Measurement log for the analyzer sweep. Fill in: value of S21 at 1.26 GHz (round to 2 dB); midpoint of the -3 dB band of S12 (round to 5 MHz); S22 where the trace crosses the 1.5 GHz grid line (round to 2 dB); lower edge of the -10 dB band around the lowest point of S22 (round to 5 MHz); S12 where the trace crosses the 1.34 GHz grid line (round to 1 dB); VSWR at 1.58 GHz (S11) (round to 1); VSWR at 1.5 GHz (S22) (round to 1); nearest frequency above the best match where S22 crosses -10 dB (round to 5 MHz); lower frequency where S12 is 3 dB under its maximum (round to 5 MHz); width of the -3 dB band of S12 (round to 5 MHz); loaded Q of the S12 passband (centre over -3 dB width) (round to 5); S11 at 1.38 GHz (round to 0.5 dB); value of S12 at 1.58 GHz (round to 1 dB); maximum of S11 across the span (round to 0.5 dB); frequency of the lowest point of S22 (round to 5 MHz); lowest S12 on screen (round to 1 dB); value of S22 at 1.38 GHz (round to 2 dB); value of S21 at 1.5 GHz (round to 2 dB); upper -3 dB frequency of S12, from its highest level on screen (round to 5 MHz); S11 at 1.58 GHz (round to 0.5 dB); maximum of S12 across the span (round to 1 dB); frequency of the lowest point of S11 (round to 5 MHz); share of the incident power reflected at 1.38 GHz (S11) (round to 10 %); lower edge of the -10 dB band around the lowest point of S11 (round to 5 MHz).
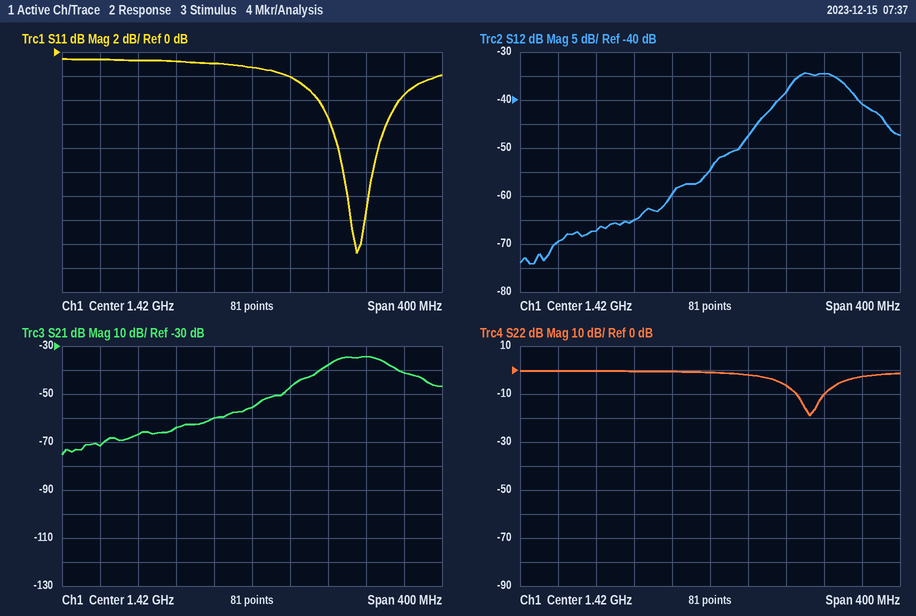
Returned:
-72 dB
1.535 GHz
-6 dB
1.510 GHz
-65 dB
5
3
1.540 GHz
1.505 GHz
60 MHz
25
-1.0 dB
-41 dB
-0.5 dB
1.525 GHz
-74 dB
0 dB
-38 dB
1.565 GHz
-3.5 dB
-34 dB
1.530 GHz
80 %
1.515 GHz
